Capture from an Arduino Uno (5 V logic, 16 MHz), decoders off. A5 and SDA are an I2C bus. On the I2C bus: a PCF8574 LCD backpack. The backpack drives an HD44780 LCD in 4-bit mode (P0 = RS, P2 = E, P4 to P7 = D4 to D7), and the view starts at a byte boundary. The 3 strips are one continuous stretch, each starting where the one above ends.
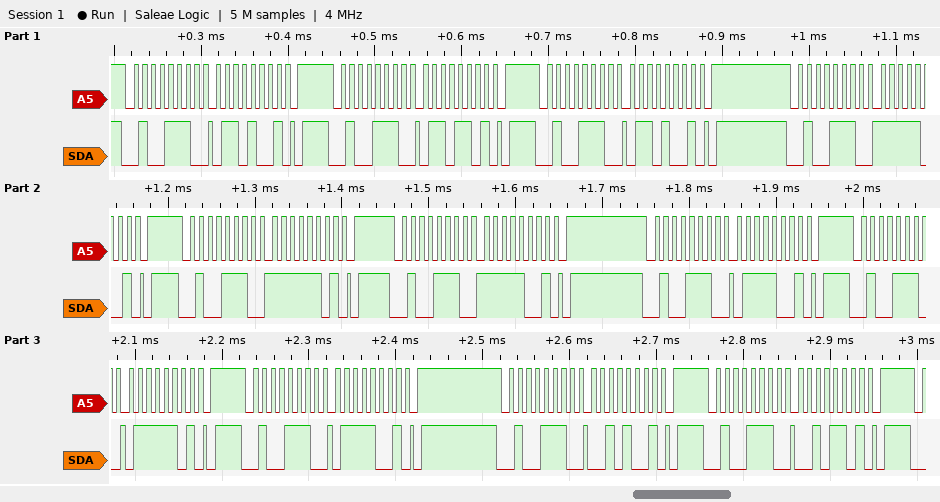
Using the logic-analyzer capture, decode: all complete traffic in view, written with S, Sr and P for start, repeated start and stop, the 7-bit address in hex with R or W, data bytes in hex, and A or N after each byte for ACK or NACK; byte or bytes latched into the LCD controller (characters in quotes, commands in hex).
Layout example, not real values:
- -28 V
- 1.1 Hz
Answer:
- S 27W A 69 A P S 27W A 6D A P S 27W A 69 A P S 27W A F9 A P S 27W A FD A P S 27W A F9 A P S 27W A 79 A P S 27W A 7D A P S 27W A 79 A P S 27W A 29 A P S 27W A 2D A P
- 'o'
